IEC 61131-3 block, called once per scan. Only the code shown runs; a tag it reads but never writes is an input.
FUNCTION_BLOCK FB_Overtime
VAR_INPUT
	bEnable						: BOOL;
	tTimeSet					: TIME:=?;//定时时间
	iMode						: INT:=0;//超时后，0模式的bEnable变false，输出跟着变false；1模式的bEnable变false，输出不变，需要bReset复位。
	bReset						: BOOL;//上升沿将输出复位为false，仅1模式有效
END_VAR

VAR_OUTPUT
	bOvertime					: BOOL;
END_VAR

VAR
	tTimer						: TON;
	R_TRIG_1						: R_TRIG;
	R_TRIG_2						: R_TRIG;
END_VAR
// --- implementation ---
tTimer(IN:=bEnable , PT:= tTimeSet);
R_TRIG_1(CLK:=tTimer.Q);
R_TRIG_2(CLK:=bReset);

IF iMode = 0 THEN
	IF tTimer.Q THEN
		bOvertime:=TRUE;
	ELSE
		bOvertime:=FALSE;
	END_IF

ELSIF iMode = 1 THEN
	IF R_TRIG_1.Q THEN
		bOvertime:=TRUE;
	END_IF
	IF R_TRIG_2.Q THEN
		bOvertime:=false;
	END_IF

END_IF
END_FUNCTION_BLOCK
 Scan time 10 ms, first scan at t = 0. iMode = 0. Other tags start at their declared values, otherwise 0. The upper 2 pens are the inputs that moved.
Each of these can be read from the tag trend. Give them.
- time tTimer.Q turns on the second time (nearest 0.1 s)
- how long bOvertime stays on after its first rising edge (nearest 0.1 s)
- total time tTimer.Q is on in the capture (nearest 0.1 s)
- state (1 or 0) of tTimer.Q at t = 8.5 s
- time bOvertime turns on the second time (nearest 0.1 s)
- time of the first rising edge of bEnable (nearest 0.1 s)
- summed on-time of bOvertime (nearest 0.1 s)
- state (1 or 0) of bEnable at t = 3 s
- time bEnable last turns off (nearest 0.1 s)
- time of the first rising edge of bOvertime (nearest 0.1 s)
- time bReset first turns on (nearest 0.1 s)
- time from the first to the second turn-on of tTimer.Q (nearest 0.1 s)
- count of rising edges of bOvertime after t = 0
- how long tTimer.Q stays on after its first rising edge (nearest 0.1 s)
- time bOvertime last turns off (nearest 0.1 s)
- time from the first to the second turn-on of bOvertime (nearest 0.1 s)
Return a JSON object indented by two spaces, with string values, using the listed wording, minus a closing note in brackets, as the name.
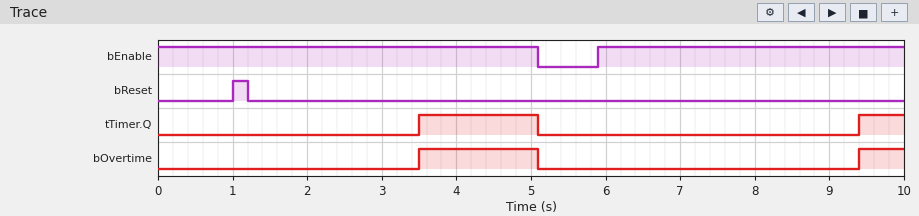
{
  "time tTimer.Q turns on the second time": "9.4 s",
  "how long bOvertime stays on after its first rising edge": "1.6 s",
  "total time tTimer.Q is on in the capture": "2.2 s",
  "state (1 or 0) of tTimer.Q at t = 8.5 s": "0",
  "time bOvertime turns on the second time": "9.4 s",
  "time of the first rising edge of bEnable": "5.9 s",
  "summed on-time of bOvertime": "2.2 s",
  "state (1 or 0) of bEnable at t = 3 s": "1",
  "time bEnable last turns off": "5.1 s",
  "time of the first rising edge of bOvertime": "3.5 s",
  "time bReset first turns on": "1.0 s",
  "time from the first to the second turn-on of tTimer.Q": "5.9 s",
  "count of rising edges of bOvertime after t = 0": "2",
  "how long tTimer.Q stays on after its first rising edge": "1.6 s",
  "time bOvertime last turns off": "5.1 s",
  "time from the first to the second turn-on of bOvertime": "5.9 s"
}
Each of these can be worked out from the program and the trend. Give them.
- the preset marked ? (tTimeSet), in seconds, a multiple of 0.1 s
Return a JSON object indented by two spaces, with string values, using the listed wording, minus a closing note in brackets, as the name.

{
  "the preset marked ? (tTimeSet), in seconds, a multiple of 0.1 s": "3.5 s"
}
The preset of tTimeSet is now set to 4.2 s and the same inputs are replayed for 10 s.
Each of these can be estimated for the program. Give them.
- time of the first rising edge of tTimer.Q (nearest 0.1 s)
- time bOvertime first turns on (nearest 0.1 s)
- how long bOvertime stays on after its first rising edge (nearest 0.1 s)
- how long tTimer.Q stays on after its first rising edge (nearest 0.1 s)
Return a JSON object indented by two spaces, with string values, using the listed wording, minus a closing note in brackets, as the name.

{
  "time of the first rising edge of tTimer.Q": "4.2 s",
  "time bOvertime first turns on": "4.2 s",
  "how long bOvertime stays on after its first rising edge": "0.9 s",
  "how long tTimer.Q stays on after its first rising edge": "0.9 s"
}
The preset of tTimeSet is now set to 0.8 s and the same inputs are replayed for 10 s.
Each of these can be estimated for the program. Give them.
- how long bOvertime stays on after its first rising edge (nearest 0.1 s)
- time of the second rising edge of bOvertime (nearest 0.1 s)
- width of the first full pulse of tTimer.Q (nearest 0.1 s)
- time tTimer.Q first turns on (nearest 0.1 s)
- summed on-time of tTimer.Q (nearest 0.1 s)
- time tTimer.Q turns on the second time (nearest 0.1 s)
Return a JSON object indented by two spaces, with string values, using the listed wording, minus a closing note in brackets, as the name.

{
  "how long bOvertime stays on after its first rising edge": "4.3 s",
  "time of the second rising edge of bOvertime": "6.7 s",
  "width of the first full pulse of tTimer.Q": "4.3 s",
  "time tTimer.Q first turns on": "0.8 s",
  "summed on-time of tTimer.Q": "7.6 s",
  "time tTimer.Q turns on the second time": "6.7 s"
}
